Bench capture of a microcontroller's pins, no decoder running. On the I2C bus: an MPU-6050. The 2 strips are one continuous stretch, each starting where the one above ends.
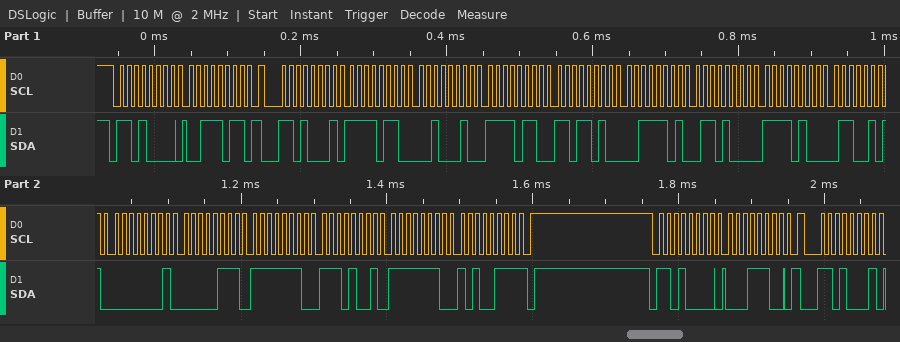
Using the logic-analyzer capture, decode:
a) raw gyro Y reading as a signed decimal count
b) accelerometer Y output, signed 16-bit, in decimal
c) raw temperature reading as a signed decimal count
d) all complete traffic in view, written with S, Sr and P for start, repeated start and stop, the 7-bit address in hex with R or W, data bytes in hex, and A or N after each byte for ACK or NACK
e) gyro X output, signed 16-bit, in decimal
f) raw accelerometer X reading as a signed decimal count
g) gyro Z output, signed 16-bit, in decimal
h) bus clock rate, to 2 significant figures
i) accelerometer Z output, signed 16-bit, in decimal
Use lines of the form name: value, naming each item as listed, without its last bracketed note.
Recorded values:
raw gyro Y reading as a signed decimal count: -279
accelerometer Y output, signed 16-bit, in decimal: -2342
raw temperature reading as a signed decimal count: -2971
all complete traffic in view, written with S, Sr and P for start, repeated start and stop, the 7-bit address in hex with R or W, data bytes in hex, and A or N after each byte for ACK or NACK: S 68W A 3B A Sr 68R A F6 A 22 A F6 A DA A 3D A 68 A F4 A 65 A 01 A 07 A FE A E9 A FE A A7 N P S 68W A 1C A Sr 68R A
gyro X output, signed 16-bit, in decimal: 263
raw accelerometer X reading as a signed decimal count: -2526
gyro Z output, signed 16-bit, in decimal: -345
bus clock rate, to 2 significant figures: 100 kHz
accelerometer Z output, signed 16-bit, in decimal: 15720
